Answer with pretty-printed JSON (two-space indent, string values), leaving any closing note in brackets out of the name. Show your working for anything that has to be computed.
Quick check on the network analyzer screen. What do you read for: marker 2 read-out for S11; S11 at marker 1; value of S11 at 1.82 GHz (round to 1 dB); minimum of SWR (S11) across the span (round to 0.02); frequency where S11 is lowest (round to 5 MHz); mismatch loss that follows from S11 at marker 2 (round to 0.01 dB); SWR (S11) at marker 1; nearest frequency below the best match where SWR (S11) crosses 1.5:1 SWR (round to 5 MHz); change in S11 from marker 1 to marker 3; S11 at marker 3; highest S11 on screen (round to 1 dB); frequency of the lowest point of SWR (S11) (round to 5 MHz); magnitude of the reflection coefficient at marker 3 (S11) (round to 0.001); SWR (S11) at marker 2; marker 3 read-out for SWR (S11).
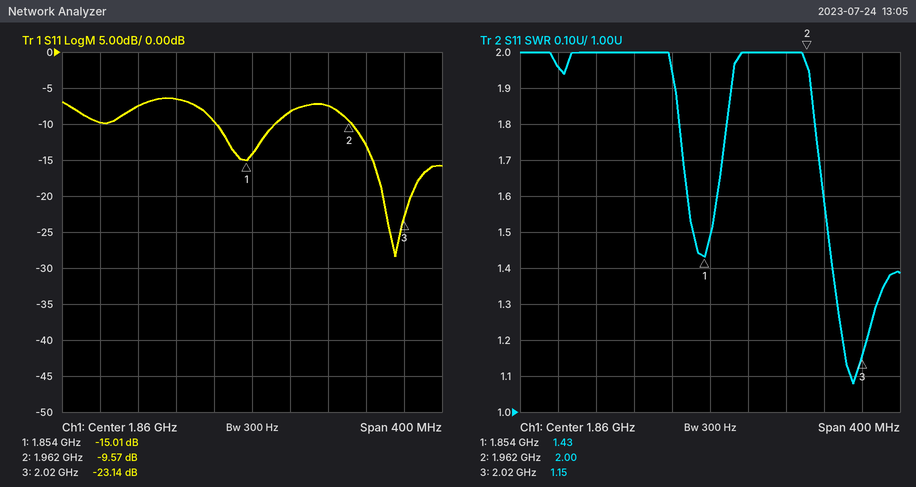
{
  "marker 2 read-out for S11": "-9.57 dB",
  "S11 at marker 1": "-15.01 dB",
  "value of S11 at 1.82 GHz": "-10 dB",
  "minimum of SWR (S11) across the span": "1.08",
  "frequency where S11 is lowest": "2.010 GHz",
  "mismatch loss that follows from S11 at marker 2": "−10 log10(1 − 10^(-9.57/10)) ≈ 0.51 dB",
  "SWR (S11) at marker 1": "1.43",
  "nearest frequency below the best match where SWR (S11) crosses 1.5:1 SWR": "1.985 GHz",
  "change in S11 from marker 1 to marker 3": "-23.14 − (-15.01) = -8.13 dB",
  "S11 at marker 3": "-23.14 dB",
  "highest S11 on screen": "-6 dB",
  "frequency of the lowest point of SWR (S11)": "2.010 GHz",
  "magnitude of the reflection coefficient at marker 3 (S11)": "10^(-23.14/20) ≈ 0.070",
  "SWR (S11) at marker 2": "2.00",
  "marker 3 read-out for SWR": "1.15"
}
